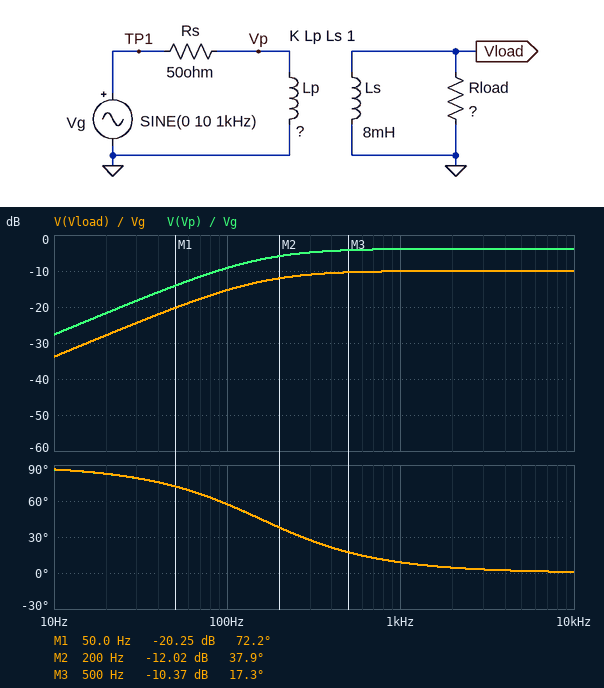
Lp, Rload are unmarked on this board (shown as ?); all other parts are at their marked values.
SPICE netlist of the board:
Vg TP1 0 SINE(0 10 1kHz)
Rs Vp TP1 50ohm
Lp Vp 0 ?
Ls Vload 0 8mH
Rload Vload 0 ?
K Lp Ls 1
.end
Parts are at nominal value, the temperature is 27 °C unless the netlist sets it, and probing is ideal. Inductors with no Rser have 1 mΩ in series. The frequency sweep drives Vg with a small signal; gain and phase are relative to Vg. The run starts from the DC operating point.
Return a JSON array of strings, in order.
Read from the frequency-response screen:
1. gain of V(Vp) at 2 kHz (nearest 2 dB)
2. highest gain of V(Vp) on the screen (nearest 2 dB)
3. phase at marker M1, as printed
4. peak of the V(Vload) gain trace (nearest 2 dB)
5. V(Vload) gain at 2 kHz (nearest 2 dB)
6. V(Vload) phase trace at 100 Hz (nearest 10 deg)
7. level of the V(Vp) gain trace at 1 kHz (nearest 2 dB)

["-4 dB", "-4 dB", "72.2 deg", "-10 dB", "-10 dB", "60 deg", "-4 dB"]
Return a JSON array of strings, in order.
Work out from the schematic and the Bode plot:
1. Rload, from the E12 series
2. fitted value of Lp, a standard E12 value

["22 Ω", "33 mH"]
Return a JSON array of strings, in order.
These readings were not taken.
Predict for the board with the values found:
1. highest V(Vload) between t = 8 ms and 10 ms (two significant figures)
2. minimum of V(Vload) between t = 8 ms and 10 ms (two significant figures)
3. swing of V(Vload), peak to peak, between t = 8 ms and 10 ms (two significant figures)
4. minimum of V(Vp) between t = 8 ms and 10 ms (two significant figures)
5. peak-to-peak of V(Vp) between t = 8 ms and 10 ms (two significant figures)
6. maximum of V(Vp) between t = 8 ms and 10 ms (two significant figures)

["3.1 V", "-3.1 V", "6.3 V", "-6.4 V", "13 V", "6.4 V"]
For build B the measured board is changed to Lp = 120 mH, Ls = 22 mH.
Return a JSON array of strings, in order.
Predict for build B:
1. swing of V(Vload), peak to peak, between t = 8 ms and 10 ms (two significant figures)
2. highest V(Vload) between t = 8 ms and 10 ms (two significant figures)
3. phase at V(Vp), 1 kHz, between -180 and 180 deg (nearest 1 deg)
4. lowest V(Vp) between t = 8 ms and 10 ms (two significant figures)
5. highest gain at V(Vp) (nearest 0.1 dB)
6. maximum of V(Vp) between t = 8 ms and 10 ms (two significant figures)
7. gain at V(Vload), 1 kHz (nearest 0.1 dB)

["6.0 V", "3.0 V", "3 deg", "-7.1 V", "-3.0 dB", "7.0 V", "-10.4 dB"]
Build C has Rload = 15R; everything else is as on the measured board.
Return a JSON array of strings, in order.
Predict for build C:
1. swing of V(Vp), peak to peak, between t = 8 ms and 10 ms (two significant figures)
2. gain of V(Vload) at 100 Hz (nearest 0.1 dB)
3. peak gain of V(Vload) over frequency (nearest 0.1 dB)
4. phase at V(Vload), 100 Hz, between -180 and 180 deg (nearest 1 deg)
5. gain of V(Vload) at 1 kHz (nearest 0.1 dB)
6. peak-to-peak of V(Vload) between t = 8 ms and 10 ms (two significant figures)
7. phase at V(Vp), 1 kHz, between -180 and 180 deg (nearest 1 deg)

["11 V", "-15.7 dB", "-11.3 dB", "53 deg", "-11.4 dB", "5.4 V", "8 deg"]
